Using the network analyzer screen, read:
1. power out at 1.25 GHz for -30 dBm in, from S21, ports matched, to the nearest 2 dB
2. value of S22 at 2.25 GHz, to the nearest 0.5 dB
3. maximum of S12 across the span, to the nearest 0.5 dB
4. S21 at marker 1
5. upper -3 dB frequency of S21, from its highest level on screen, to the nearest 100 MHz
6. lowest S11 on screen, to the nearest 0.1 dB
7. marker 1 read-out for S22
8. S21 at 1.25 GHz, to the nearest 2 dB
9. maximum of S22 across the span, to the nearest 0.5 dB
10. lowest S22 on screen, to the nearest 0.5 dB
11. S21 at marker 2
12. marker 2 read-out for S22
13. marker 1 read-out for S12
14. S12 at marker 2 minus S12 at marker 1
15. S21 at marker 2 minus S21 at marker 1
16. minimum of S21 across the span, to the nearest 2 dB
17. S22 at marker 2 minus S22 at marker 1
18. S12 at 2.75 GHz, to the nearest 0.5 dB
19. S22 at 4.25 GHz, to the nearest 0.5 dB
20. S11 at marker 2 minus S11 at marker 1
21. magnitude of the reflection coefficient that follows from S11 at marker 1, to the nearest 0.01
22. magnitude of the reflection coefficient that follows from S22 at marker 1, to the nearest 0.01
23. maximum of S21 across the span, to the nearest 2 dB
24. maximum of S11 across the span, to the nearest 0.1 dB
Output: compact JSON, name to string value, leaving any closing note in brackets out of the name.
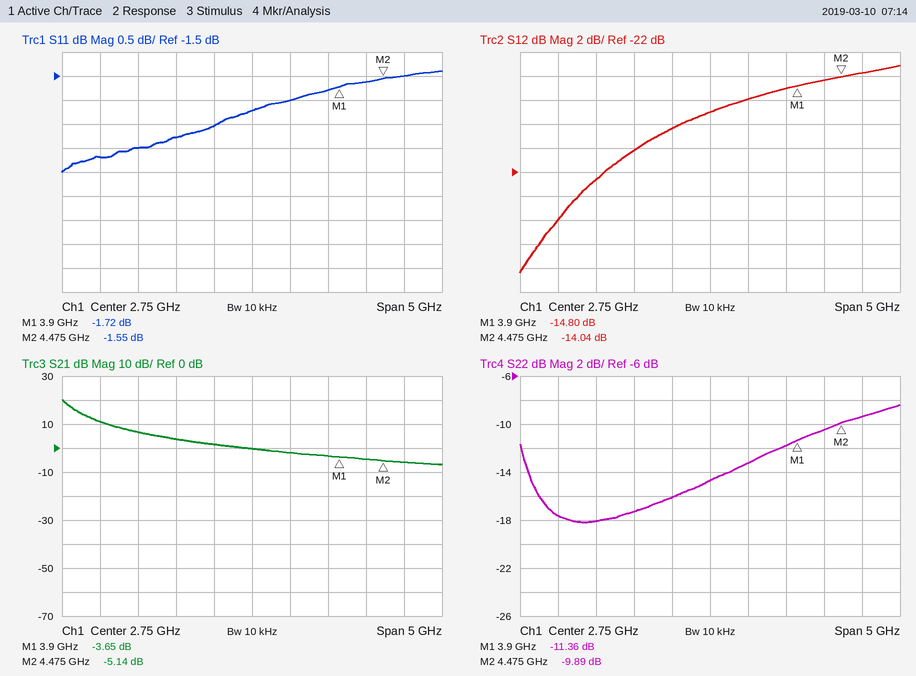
{"power out at 1.25 GHz for -30 dBm in, from S21, ports matched, to the nearest 2 dB": "-24 dBm", "value of S22 at 2.25 GHz, to the nearest 0.5 dB": "-16.0 dB", "maximum of S12 across the span, to the nearest 0.5 dB": "-13.0 dB", "S21 at marker 1": "-3.65 dB", "upper -3 dB frequency of S21, from its highest level on screen, to the nearest 100 MHz": "400 MHz", "lowest S11 on screen, to the nearest 0.1 dB": "-3.5 dB", "marker 1 read-out for S22": "-11.36 dB", "S21 at 1.25 GHz, to the nearest 2 dB": "6 dB", "maximum of S22 across the span, to the nearest 0.5 dB": "-8.5 dB", "lowest S22 on screen, to the nearest 0.5 dB": "-18.0 dB", "S21 at marker 2": "-5.14 dB", "marker 2 read-out for S22": "-9.89 dB", "marker 1 read-out for S12": "-14.80 dB", "S12 at marker 2 minus S12 at marker 1": "0.76 dB", "S21 at marker 2 minus S21 at marker 1": "-1.49 dB", "minimum of S21 across the span, to the nearest 2 dB": "-6 dB", "S22 at marker 2 minus S22 at marker 1": "1.47 dB", "S12 at 2.75 GHz, to the nearest 0.5 dB": "-17.0 dB", "S22 at 4.25 GHz, to the nearest 0.5 dB": "-10.5 dB", "S11 at marker 2 minus S11 at marker 1": "0.17 dB", "magnitude of the reflection coefficient that follows from S11 at marker 1, to the nearest 0.01": "0.82", "magnitude of the reflection coefficient that follows from S22 at marker 1, to the nearest 0.01": "0.27", "maximum of S21 across the span, to the nearest 2 dB": "20 dB", "maximum of S11 across the span, to the nearest 0.1 dB": "-1.4 dB"}
